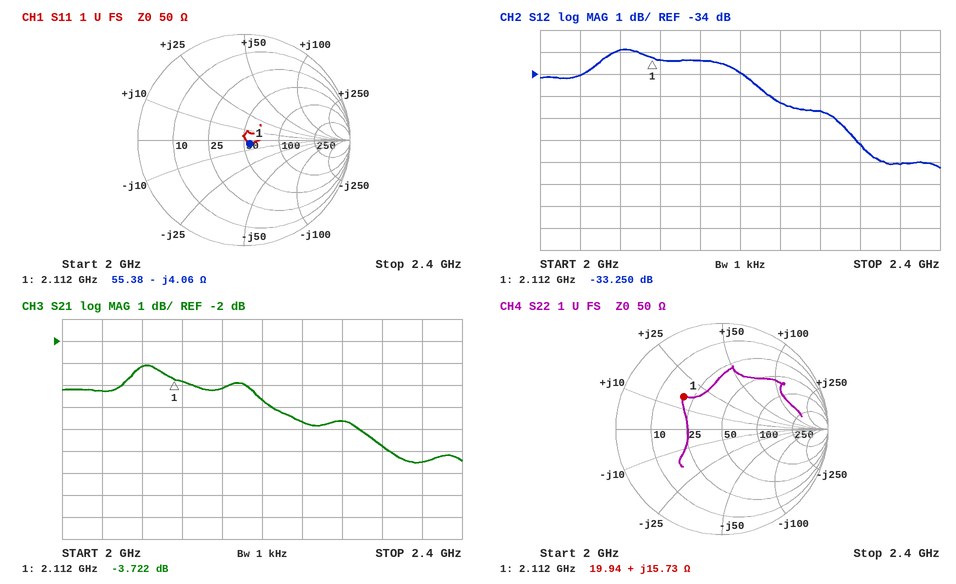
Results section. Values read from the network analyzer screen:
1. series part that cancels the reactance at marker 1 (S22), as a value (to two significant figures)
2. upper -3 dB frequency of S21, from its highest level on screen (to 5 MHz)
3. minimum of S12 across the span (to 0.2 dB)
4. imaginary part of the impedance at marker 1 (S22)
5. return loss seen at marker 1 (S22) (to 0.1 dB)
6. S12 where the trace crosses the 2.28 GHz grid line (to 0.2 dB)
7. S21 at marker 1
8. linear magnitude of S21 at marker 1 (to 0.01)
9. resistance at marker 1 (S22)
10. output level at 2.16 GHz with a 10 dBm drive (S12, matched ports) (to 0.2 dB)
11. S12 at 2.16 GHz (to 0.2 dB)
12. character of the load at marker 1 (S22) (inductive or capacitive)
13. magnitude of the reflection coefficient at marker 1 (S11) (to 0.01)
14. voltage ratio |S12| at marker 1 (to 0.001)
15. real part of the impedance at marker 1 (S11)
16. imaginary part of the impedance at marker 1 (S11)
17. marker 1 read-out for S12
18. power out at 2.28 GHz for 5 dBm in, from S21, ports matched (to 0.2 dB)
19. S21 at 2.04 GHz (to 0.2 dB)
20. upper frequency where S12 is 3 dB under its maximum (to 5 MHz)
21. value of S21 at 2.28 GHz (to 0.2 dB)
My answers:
4.8 pF
2.300 GHz
-38.2 dB
+15.73 Ω
6.5 dB
-35.6 dB
-3.722 dB
0.65
19.94 Ω
-23.4 dBm
-33.4 dB
inductive
0.06
0.022
55.38 Ω
-4.06 Ω
-33.250 dB
-0.6 dBm
-4.2 dB
2.290 GHz
-5.6 dB
